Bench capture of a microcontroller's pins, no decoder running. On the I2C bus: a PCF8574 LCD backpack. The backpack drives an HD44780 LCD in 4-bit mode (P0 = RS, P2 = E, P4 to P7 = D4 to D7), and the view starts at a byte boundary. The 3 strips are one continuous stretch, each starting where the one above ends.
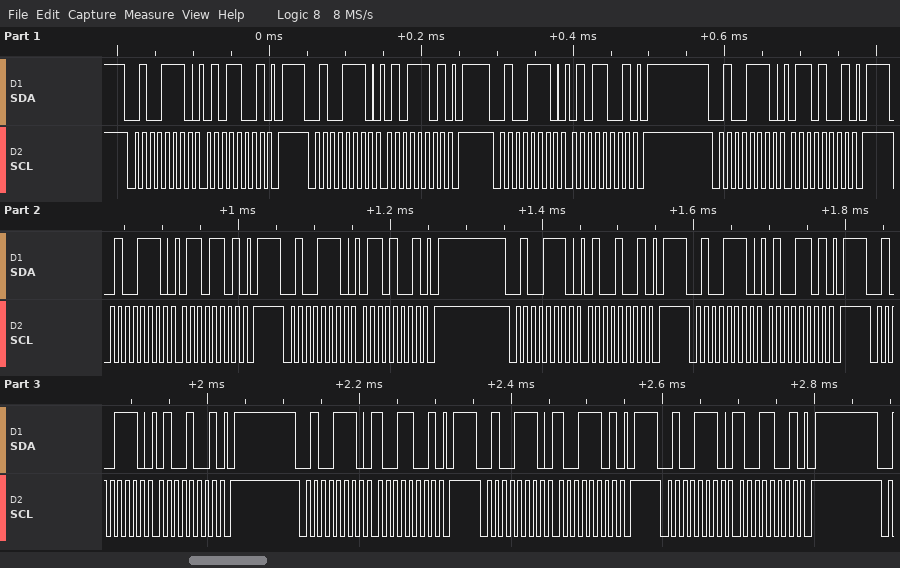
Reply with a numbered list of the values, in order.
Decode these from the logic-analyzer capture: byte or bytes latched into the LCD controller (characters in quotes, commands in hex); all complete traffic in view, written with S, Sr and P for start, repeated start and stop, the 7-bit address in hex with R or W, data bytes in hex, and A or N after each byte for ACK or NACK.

1. 'V' 'I'
2. S 27W A 59 A P S 27W A 5D A P S 27W A 59 A P S 27W A 69 A P S 27W A 6D A P S 27W A 69 A P S 27W A 49 A P S 27W A 4D A P S 27W A 49 A P S 27W A 99 A P S 27W A 9D A P S 27W A 99 A P
